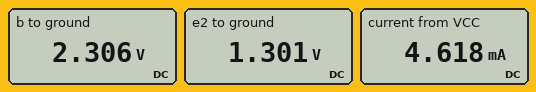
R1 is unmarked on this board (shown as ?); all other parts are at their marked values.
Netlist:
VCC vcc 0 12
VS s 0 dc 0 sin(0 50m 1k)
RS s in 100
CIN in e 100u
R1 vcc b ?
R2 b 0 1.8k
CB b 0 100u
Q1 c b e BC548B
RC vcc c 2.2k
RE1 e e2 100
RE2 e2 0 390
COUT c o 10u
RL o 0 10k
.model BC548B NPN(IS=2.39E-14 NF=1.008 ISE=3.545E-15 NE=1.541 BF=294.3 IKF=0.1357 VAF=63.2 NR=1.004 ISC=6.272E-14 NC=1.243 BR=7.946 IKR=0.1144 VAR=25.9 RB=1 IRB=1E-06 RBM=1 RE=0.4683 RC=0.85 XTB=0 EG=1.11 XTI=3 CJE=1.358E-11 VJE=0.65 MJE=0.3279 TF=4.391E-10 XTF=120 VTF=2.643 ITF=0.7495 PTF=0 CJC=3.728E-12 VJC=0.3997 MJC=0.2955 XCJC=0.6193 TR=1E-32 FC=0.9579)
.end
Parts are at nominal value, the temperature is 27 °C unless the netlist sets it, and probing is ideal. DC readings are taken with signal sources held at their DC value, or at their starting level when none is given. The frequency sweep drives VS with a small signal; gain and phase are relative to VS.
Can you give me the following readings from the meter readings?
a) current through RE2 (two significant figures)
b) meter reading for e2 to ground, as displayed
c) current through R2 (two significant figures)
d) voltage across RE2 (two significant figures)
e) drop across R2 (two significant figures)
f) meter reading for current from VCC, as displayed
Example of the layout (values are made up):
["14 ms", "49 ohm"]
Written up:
["3.3 mA", "1.301 V", "1.3 mA", "1.3 V", "2.3 V", "4.618 mA"]
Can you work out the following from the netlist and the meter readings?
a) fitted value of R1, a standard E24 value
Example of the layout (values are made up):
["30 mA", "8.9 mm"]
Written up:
["7.5 kΩ"]
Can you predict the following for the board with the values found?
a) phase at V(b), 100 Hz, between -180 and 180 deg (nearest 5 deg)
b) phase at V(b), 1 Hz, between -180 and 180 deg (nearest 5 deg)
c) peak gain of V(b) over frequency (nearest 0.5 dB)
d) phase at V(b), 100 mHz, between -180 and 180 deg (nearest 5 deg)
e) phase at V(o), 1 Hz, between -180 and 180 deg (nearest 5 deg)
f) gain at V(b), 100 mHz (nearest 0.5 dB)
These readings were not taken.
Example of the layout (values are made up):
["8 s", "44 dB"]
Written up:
["-80 deg", "45 deg", "-49.0 dB", "85 deg", "140 deg", "-69.0 dB"]
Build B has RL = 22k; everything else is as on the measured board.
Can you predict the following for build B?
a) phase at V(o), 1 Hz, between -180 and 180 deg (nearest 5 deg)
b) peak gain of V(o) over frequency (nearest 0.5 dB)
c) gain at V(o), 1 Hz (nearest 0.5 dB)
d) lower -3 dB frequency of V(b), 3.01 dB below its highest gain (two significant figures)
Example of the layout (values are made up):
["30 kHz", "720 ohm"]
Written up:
["120 deg", "25.0 dB", "0 dB", "960 mHz"]
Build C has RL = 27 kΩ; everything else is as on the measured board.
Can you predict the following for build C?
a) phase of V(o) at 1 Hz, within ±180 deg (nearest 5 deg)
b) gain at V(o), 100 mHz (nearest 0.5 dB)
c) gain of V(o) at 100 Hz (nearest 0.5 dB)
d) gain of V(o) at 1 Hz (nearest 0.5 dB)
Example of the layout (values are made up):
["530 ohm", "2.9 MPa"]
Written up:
["115 deg", "-33.0 dB", "25.0 dB", "0.5 dB"]
